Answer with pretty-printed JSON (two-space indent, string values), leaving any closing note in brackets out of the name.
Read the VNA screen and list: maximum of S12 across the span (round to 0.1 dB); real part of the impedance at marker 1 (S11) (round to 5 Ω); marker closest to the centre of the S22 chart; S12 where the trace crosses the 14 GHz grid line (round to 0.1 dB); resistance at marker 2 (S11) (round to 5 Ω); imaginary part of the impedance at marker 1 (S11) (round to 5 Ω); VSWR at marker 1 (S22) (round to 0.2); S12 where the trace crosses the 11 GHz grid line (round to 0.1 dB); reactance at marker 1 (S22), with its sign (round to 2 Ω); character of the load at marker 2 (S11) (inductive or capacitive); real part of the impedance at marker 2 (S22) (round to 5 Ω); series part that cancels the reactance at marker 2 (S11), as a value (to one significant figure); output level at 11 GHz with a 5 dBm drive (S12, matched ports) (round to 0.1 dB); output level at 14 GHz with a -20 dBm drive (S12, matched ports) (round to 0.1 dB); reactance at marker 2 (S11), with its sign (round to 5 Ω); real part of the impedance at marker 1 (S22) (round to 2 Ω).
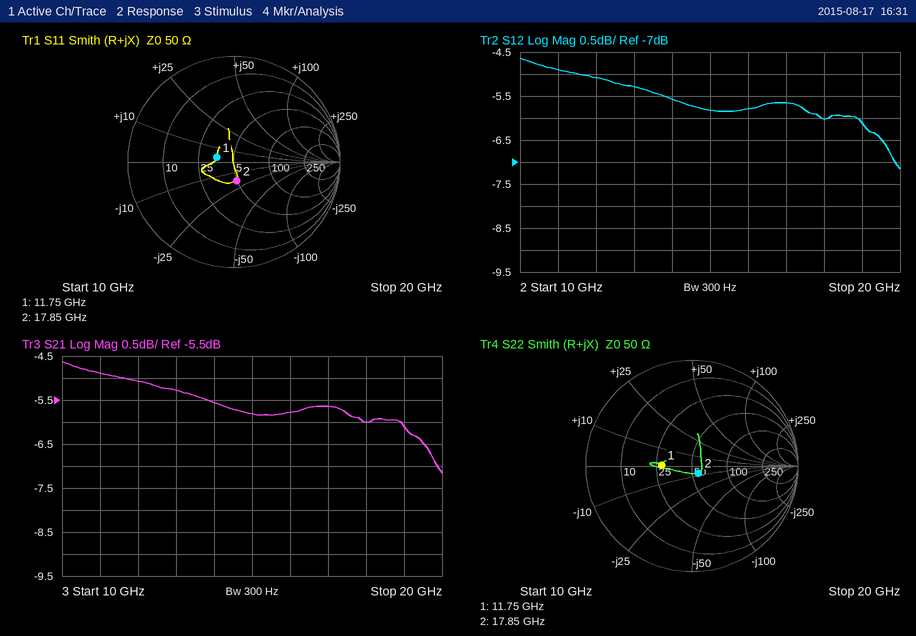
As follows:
{
  "maximum of S12 across the span": "-4.6 dB",
  "real part of the impedance at marker 1 (S11)": "35 Ω",
  "marker closest to the centre of the S22 chart": "marker 2",
  "S12 where the trace crosses the 14 GHz grid line": "-5.6 dB",
  "resistance at marker 2 (S11)": "50 Ω",
  "imaginary part of the impedance at marker 1 (S11)": "+5 Ω",
  "VSWR at marker 1 (S22)": "1.8",
  "S12 where the trace crosses the 11 GHz grid line": "-4.9 dB",
  "reactance at marker 1 (S22), with its sign": "0 Ω",
  "character of the load at marker 2 (S11)": "capacitive",
  "real part of the impedance at marker 2 (S22)": "55 Ω",
  "series part that cancels the reactance at marker 2 (S11), as a value": "200 pH",
  "output level at 11 GHz with a 5 dBm drive (S12, matched ports)": "0.1 dBm",
  "output level at 14 GHz with a -20 dBm drive (S12, matched ports)": "-25.6 dBm",
  "reactance at marker 2 (S11), with its sign": "-20 Ω",
  "real part of the impedance at marker 1 (S22)": "28 Ω"
}
